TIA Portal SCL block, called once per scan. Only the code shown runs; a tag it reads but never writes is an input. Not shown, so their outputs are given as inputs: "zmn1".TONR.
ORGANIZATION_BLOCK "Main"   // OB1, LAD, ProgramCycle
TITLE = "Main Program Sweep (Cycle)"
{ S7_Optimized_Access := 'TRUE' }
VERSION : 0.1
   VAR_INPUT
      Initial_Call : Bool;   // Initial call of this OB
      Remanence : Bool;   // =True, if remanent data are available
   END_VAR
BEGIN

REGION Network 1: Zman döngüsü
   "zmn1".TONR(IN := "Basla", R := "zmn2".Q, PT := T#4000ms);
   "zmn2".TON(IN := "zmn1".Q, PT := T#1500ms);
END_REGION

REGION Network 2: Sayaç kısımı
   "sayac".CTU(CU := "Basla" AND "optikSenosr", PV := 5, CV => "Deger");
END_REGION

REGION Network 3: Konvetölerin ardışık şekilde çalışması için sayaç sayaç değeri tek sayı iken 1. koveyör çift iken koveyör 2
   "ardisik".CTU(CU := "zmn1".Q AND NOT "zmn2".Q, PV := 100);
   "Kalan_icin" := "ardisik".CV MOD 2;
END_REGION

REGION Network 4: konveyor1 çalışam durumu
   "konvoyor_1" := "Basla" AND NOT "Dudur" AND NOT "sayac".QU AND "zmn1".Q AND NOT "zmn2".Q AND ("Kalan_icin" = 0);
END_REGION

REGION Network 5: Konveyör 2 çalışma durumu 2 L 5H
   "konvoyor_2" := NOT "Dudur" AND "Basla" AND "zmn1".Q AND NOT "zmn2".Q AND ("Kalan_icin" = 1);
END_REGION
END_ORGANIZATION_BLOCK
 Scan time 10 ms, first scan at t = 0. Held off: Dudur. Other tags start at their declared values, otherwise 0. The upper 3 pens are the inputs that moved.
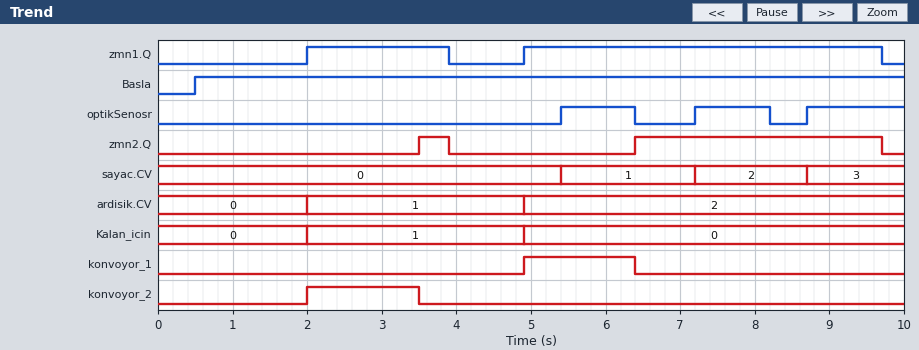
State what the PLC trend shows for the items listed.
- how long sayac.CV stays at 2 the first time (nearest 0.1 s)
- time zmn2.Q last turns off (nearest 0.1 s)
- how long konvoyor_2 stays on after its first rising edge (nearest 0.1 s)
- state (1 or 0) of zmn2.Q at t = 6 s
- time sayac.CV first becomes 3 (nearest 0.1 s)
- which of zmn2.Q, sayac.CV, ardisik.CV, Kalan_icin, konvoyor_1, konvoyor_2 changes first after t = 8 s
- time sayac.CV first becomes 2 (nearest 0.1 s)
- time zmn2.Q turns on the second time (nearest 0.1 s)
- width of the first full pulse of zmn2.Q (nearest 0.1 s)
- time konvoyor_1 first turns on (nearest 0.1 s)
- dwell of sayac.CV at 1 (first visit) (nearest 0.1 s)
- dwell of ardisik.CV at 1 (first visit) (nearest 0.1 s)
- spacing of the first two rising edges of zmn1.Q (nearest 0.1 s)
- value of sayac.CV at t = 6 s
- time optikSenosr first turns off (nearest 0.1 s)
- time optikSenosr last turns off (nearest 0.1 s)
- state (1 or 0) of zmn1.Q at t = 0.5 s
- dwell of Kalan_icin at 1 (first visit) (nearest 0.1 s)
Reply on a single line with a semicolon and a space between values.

1.5 s; 9.7 s; 1.5 s; 0; 8.7 s; sayac.CV; 7.2 s; 6.4 s; 0.4 s; 4.9 s; 1.8 s; 2.9 s; 2.9 s; 1; 6.4 s; 8.2 s; 0; 2.9 s
